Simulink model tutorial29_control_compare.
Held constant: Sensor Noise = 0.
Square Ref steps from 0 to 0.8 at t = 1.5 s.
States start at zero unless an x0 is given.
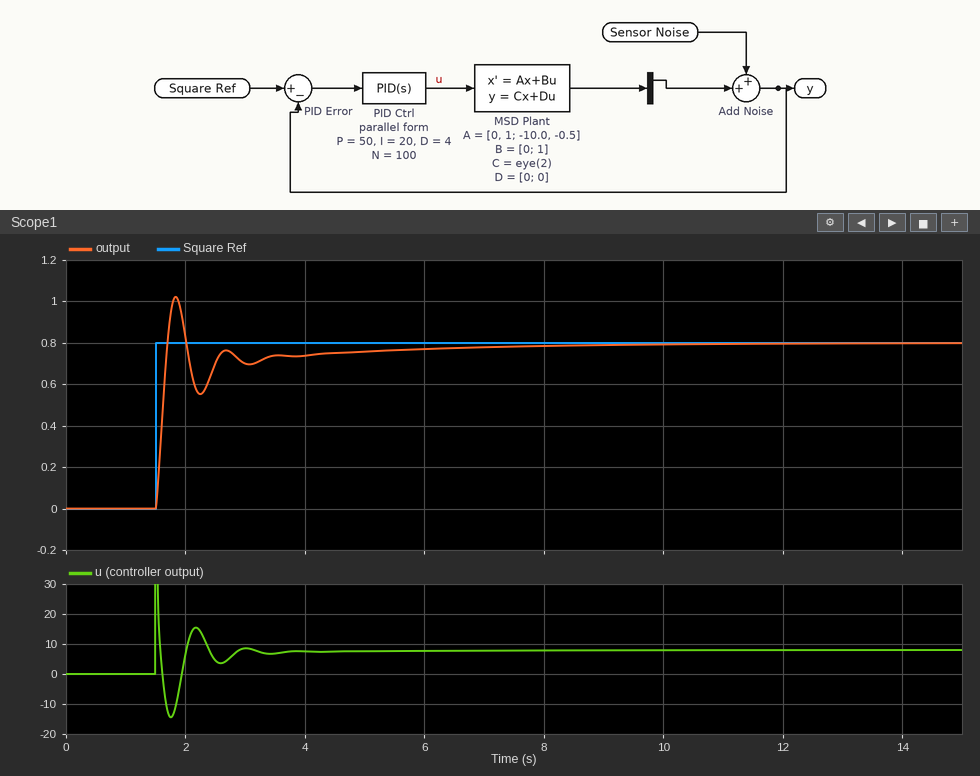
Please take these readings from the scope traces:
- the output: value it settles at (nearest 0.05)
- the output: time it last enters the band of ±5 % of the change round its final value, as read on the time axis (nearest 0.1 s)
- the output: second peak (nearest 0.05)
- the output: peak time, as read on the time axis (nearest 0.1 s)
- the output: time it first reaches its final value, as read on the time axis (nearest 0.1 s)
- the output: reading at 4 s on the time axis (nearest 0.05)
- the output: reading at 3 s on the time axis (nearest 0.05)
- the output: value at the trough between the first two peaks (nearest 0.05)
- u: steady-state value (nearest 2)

0.80
5.1 s
0.75
1.8 s
1.7 s
0.75
0.70
0.55
8
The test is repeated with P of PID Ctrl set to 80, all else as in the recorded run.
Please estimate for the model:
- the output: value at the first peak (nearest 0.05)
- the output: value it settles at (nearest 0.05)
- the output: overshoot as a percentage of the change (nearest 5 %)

1.10
0.80
40 %
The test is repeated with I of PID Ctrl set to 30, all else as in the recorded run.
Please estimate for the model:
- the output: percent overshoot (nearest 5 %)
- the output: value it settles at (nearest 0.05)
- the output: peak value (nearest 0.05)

30 %
0.80
1.05
